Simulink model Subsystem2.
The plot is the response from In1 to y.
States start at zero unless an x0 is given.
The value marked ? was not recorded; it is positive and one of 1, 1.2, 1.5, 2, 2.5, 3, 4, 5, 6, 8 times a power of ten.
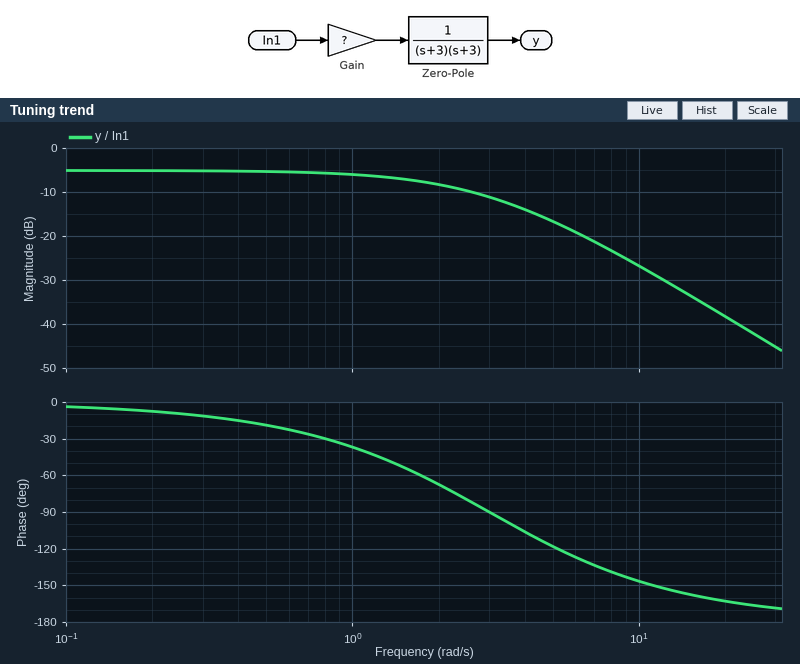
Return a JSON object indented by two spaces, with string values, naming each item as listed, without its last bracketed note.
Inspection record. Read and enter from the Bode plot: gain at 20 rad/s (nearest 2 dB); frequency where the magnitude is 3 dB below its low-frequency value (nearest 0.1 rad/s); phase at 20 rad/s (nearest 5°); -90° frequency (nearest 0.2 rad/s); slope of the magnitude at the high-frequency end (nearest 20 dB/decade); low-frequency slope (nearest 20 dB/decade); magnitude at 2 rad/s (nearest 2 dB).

{
  "gain at 20 rad/s": "-38 dB",
  "frequency where the magnitude is 3 dB below its low-frequency value": "1.9 rad/s",
  "phase at 20 rad/s": "-165°",
  "-90° frequency": "3.0 rad/s",
  "slope of the magnitude at the high-frequency end": "-40 dB/decade",
  "low-frequency slope": "0 dB/decade",
  "magnitude at 2 rad/s": "-8 dB"
}
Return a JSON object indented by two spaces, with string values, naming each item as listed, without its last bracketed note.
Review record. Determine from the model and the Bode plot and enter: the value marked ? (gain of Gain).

{
  "the value marked ?": "5"
}
